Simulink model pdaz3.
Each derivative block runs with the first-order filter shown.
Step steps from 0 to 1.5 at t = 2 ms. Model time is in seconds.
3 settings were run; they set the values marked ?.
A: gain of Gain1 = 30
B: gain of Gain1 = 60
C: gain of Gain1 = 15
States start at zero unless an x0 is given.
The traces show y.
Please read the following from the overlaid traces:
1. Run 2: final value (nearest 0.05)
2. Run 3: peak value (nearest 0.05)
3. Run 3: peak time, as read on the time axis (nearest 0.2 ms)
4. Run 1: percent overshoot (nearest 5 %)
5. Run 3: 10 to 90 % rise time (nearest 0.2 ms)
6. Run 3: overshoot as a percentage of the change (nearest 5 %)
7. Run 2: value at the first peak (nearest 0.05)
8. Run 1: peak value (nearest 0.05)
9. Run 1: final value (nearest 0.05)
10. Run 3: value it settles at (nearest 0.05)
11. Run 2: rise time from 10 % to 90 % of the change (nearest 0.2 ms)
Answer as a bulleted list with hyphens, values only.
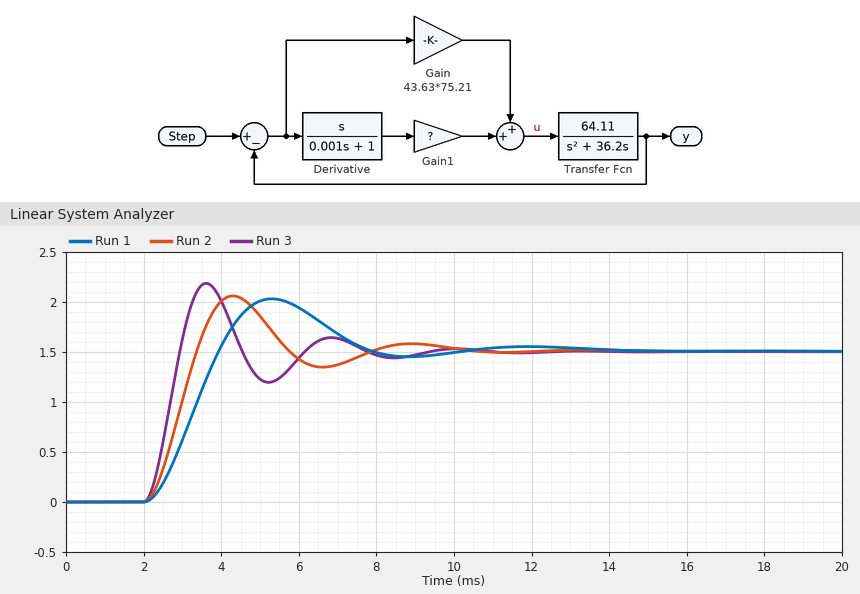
- 1.50
- 2.20
- 3.6 ms
- 35 %
- 0.6 ms
- 45 %
- 2.05
- 2.05
- 1.50
- 1.50
- 1.0 ms
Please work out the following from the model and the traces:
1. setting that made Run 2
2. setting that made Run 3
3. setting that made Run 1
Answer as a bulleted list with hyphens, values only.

- A
- B
- C
